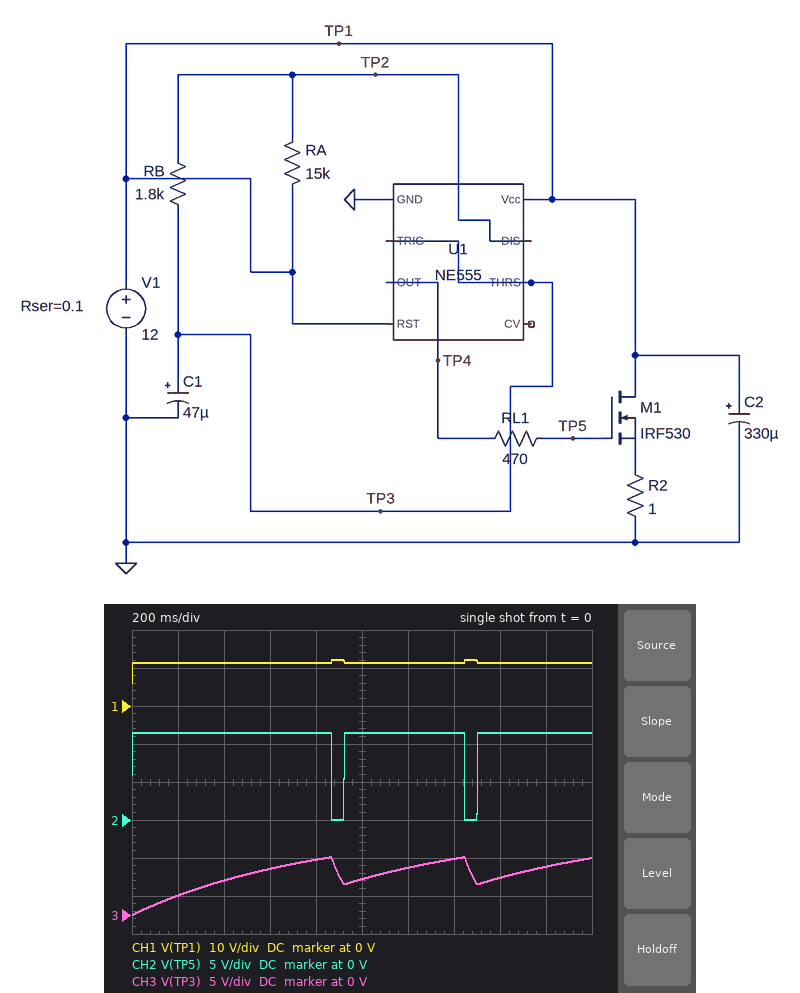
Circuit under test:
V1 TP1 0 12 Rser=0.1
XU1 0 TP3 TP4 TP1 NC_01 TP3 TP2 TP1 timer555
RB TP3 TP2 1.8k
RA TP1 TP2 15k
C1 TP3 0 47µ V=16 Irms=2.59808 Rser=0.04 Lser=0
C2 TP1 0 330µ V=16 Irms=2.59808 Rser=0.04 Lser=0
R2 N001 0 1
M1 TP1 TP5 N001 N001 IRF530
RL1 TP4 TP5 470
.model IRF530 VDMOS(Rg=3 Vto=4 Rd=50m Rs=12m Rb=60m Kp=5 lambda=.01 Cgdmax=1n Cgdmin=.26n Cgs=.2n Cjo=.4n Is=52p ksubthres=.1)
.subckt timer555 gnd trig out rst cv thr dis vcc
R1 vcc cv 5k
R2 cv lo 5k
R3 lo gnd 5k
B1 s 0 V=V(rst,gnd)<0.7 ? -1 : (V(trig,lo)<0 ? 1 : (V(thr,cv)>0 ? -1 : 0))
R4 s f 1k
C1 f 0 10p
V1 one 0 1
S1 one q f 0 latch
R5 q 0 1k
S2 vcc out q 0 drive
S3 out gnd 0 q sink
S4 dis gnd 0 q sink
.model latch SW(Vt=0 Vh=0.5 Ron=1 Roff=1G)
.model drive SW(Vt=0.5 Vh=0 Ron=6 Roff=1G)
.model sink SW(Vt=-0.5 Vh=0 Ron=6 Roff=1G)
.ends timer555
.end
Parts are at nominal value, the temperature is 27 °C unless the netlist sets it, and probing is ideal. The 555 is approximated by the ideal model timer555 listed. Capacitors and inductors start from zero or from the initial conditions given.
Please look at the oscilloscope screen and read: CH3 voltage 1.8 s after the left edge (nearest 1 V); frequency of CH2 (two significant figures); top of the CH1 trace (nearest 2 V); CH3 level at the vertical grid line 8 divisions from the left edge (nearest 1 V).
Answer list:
6 V
1.7 Hz
12 V
5 V
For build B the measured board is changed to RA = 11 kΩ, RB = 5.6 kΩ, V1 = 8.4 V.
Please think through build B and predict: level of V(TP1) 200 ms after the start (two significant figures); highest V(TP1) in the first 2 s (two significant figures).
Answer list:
8.1 V
8.4 V
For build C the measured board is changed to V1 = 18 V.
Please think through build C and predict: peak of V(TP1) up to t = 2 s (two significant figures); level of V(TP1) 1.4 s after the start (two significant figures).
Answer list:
18 V
17 V
